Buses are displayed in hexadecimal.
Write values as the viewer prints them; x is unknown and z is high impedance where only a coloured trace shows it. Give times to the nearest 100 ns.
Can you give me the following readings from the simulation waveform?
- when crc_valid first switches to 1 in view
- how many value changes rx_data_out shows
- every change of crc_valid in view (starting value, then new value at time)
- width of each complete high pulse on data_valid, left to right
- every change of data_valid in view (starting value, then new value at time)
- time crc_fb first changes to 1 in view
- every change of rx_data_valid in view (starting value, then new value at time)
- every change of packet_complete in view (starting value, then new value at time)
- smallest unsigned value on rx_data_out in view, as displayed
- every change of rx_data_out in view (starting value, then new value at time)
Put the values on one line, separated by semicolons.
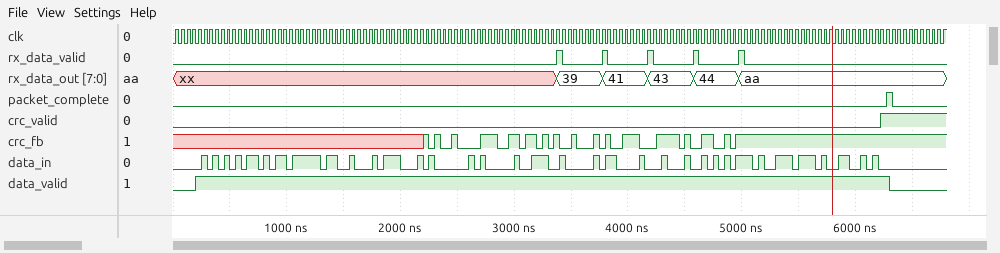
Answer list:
6200 ns; 5; 0, 1 at 6200 ns; 6100 ns; 0, 1 at 200 ns, 0 at 6300 ns; 2200 ns; 0, 1 at 3400 ns, 0 at 3400 ns, 1 at 3800 ns, 0 at 3800 ns, 1 at 4200 ns, 0 at 4200 ns, 1 at 4600 ns, 0 at 4600 ns, 1 at 5000 ns, 0 at 5000 ns; 0, 1 at 6300 ns, 0 at 6300 ns; 39; xx, 39 at 3400 ns, 41 at 3800 ns, 43 at 4200 ns, 44 at 4600 ns, aa at 5000 ns
